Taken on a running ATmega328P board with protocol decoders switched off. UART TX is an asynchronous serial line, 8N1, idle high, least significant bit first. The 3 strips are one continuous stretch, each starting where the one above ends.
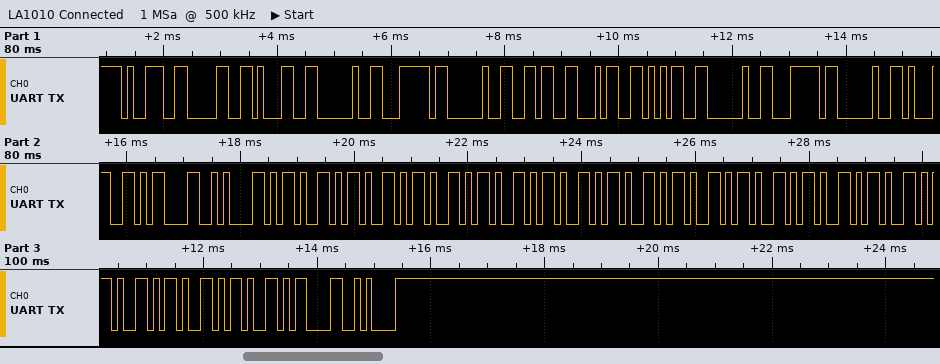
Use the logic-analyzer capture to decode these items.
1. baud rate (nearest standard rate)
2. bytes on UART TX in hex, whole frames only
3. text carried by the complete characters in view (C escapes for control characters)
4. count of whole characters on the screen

9600 baud
39 30 31 20 7C 20 36 34 35 20 7C 20 31 0D 0A 2D 2D 2D 2D 2D 2D 2D 2D 2D 2D 2D 2D 2D 0D 0A
"901 | 645 | 1\r\n-------------\r\n"
30
